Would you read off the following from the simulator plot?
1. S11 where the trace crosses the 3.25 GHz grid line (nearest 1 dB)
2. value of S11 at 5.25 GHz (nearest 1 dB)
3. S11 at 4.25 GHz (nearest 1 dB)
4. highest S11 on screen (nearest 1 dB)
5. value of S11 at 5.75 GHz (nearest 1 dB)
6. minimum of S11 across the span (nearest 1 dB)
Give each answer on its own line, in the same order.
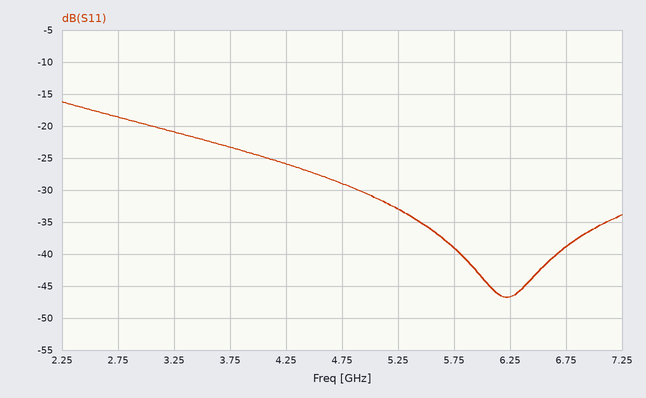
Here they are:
-21 dB
-33 dB
-26 dB
-16 dB
-39 dB
-47 dB
